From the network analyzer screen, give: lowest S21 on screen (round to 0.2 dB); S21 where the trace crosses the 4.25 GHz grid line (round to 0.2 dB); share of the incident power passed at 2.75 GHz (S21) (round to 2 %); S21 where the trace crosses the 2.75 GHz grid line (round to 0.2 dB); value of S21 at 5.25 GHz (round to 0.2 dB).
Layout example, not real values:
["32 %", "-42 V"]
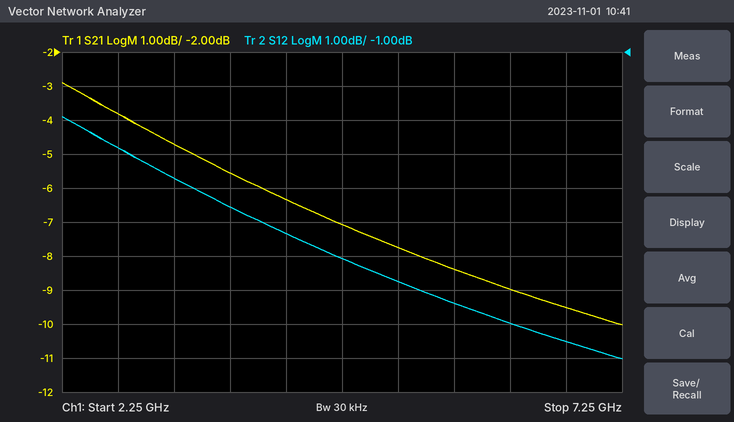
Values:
["-10.0 dB", "-6.4 dB", "42 %", "-3.8 dB", "-7.8 dB"]
